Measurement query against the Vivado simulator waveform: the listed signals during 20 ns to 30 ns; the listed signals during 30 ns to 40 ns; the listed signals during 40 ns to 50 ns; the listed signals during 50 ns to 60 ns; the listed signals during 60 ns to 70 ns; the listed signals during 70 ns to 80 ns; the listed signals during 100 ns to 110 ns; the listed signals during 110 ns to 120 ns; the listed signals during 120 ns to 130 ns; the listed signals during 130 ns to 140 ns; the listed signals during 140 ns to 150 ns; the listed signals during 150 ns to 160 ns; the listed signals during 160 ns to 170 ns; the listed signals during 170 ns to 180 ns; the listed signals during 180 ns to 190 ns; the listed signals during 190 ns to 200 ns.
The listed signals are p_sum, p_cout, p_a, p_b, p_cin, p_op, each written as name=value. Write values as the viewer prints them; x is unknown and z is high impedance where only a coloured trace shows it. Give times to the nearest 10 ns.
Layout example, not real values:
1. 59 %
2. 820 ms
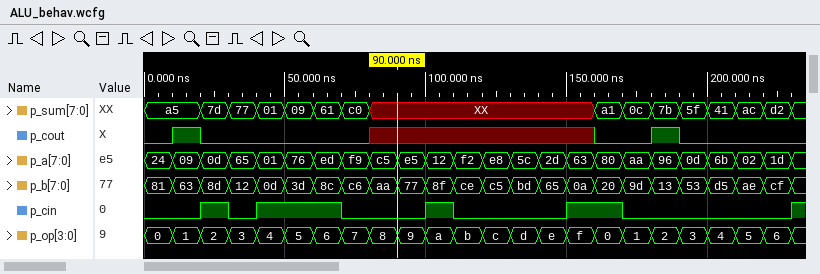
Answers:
1. p_sum=7d, p_cout=0, p_a=0d, p_b=8d, p_cin=1, p_op=2
2. p_sum=77, p_cout=0, p_a=65, p_b=12, p_cin=0, p_op=3
3. p_sum=01, p_cout=0, p_a=01, p_b=0d, p_cin=1, p_op=4
4. p_sum=09, p_cout=0, p_a=76, p_b=3d, p_cin=1, p_op=5
5. p_sum=61, p_cout=0, p_a=ed, p_b=8c, p_cin=1, p_op=6
6. p_sum=c0, p_cout=0, p_a=f9, p_b=c6, p_cin=0, p_op=7
7. p_sum=XX, p_cout=x, p_a=12, p_b=8f, p_cin=1, p_op=a
8. p_sum=XX, p_cout=x, p_a=f2, p_b=ce, p_cin=0, p_op=b
9. p_sum=XX, p_cout=x, p_a=e8, p_b=c5, p_cin=0, p_op=c
10. p_sum=XX, p_cout=x, p_a=5c, p_b=bd, p_cin=0, p_op=d
11. p_sum=XX, p_cout=x, p_a=2d, p_b=65, p_cin=0, p_op=e
12. p_sum=XX, p_cout=x, p_a=63, p_b=0a, p_cin=1, p_op=f
13. p_sum=a1, p_cout=0, p_a=80, p_b=20, p_cin=1, p_op=0
14. p_sum=0c, p_cout=0, p_a=aa, p_b=9d, p_cin=0, p_op=1
15. p_sum=7b, p_cout=1, p_a=96, p_b=13, p_cin=0, p_op=2
16. p_sum=5f, p_cout=0, p_a=0d, p_b=53, p_cin=0, p_op=3
